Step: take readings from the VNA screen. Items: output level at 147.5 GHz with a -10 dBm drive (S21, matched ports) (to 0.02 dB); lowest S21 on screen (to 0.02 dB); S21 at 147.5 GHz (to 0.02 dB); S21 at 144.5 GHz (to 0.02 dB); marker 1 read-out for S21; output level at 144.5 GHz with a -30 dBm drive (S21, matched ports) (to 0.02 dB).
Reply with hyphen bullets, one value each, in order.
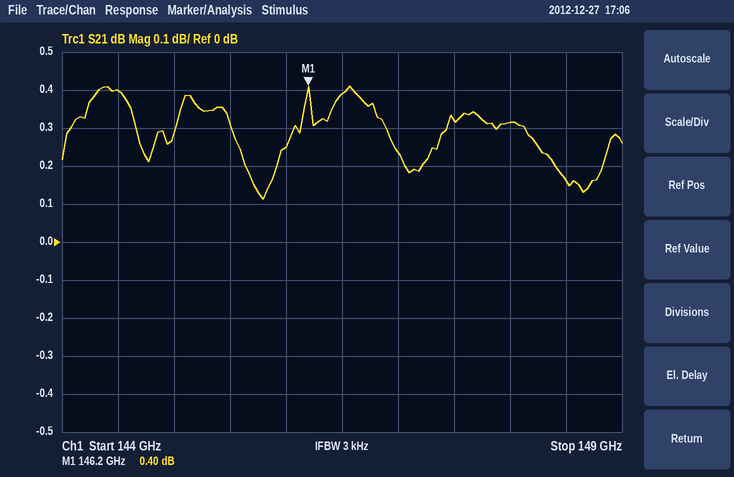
- -9.68 dBm
- 0.12 dB
- 0.32 dB
- 0.40 dB
- 0.40 dB
- -29.60 dBm
